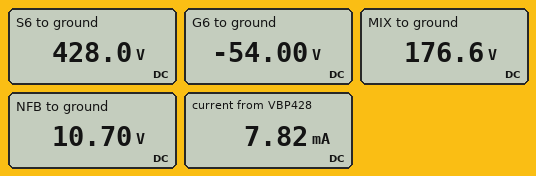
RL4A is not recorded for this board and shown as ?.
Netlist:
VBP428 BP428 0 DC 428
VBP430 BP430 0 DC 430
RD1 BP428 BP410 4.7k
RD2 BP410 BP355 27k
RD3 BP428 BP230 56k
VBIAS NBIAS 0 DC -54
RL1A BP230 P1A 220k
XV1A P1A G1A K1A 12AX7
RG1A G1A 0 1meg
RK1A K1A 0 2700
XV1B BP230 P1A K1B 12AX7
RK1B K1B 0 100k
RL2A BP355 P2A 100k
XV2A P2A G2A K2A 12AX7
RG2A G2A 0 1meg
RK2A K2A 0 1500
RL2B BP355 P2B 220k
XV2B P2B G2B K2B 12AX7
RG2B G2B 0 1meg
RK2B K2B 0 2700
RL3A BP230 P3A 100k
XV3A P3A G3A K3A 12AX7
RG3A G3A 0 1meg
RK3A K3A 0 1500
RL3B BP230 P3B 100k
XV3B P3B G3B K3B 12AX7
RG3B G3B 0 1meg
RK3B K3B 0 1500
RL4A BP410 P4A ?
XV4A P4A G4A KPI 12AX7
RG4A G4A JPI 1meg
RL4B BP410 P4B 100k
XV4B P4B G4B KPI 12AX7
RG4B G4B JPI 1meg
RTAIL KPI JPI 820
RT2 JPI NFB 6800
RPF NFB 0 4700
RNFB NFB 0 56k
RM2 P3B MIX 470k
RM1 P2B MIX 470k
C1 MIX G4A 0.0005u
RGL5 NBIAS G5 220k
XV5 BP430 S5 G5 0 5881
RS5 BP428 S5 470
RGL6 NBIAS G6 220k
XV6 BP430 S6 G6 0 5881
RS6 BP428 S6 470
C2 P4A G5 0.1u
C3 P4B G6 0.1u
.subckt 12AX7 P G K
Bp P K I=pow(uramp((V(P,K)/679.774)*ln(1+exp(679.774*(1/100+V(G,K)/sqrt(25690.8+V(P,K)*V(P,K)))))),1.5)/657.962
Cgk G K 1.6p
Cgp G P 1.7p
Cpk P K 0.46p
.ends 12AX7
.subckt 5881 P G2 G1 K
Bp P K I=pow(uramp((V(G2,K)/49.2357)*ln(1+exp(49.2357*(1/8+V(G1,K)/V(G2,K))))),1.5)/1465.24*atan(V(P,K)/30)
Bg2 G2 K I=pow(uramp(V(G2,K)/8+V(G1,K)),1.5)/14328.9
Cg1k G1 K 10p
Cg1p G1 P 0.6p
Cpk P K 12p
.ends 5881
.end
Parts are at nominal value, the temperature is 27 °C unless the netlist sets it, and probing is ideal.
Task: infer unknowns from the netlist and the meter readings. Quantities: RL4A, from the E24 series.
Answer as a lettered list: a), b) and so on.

a) 100 kΩ
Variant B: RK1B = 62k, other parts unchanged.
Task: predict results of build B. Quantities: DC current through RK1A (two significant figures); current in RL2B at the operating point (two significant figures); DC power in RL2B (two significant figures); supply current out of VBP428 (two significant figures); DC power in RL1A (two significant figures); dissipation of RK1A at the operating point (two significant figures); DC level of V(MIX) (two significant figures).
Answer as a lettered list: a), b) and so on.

a) 450 µA
b) 730 µA
c) 120 mW
d) 8.2 mA
e) 45 mW
f) 550 µW
g) 170 V
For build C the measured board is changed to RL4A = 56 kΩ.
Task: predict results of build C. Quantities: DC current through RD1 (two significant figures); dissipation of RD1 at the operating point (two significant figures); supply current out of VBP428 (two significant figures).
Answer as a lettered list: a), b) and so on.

a) 4.6 mA
b) 99 mW
c) 8.0 mA
